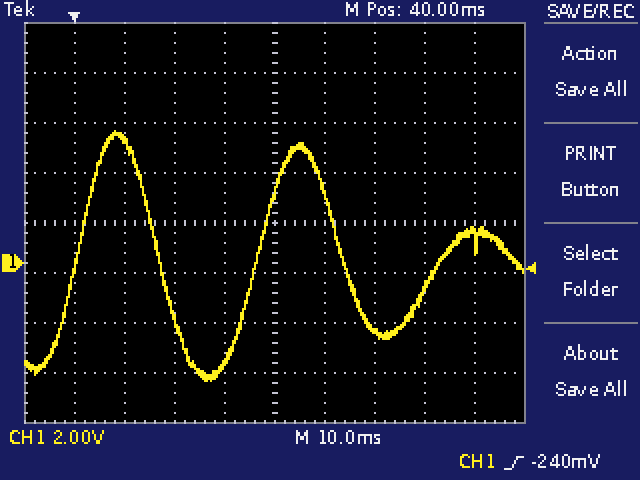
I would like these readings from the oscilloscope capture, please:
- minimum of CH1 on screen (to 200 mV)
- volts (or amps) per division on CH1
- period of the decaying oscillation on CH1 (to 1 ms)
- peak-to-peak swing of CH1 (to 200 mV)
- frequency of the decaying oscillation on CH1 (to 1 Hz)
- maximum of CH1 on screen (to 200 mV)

-4.8 V
2 V
36 ms
10.0 V
28 Hz
5.2 V
